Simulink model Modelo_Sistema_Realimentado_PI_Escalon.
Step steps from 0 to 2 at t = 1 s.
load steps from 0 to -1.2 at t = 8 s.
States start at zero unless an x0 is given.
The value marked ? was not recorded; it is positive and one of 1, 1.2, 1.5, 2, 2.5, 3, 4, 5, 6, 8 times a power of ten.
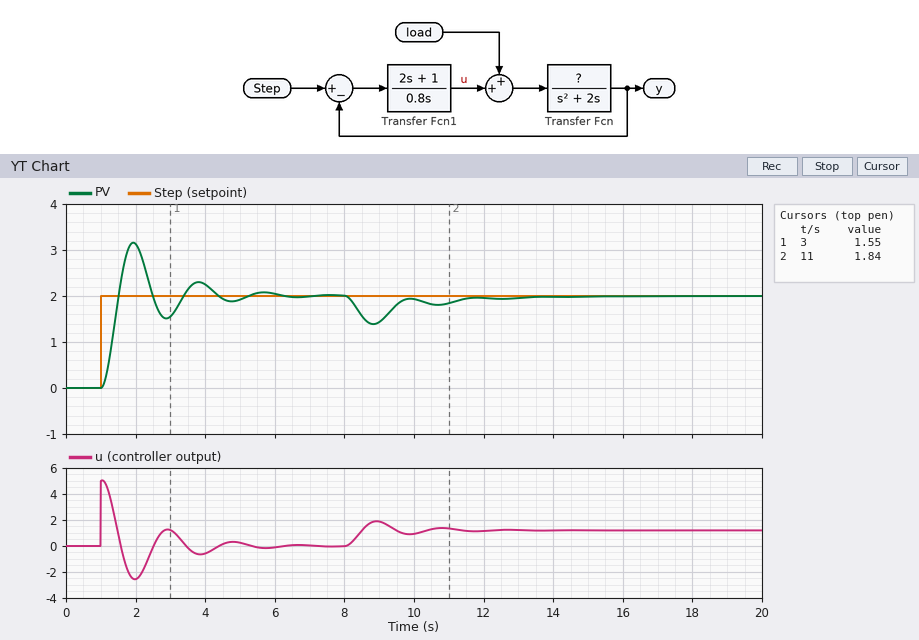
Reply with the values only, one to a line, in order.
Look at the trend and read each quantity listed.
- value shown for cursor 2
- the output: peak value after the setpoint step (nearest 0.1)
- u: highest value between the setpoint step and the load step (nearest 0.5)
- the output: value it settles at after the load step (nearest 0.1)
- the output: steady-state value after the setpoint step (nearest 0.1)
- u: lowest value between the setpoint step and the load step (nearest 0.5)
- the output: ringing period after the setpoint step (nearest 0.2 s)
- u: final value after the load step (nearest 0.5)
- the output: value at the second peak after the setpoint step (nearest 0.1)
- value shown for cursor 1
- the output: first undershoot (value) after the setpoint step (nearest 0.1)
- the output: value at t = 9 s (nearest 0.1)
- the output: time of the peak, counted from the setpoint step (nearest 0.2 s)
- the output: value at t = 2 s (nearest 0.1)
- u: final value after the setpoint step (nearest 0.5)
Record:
1.84
3.2
5.0
2.0
2.0
-2.5
1.8 s
1.0
2.3
1.55
1.5
1.4
1.0 s
3.1
0.0
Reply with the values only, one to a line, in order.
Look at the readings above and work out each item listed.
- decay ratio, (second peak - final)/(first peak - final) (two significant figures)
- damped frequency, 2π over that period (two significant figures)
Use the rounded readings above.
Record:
0.25
3.5 rad/s
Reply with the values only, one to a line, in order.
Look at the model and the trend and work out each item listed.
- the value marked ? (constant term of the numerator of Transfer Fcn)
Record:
5
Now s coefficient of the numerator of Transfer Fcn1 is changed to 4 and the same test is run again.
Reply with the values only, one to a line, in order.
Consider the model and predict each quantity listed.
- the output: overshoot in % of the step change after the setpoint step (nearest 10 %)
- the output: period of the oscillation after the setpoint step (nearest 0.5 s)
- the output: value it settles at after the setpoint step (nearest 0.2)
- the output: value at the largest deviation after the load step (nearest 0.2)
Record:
60 %
1.5 s
2.0
1.6
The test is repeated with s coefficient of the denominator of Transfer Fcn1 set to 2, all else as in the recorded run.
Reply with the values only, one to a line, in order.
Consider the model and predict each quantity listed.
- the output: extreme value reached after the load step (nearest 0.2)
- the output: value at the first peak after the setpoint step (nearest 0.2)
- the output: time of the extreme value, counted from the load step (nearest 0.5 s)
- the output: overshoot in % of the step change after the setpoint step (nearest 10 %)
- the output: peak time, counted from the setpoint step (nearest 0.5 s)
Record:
0.8
3.0
1.5 s
50 %
1.5 s
